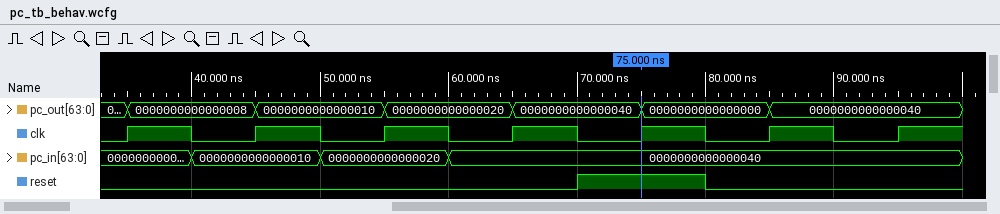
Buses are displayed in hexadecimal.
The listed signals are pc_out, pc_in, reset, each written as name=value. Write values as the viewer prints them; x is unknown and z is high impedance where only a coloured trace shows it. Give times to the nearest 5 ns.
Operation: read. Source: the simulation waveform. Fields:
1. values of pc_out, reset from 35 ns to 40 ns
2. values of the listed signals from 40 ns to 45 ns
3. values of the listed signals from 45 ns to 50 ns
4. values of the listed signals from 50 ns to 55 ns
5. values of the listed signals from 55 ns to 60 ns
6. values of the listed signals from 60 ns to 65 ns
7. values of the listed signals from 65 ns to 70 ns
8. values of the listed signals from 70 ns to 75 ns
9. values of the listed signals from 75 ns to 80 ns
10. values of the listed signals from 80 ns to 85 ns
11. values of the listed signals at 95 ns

pc_out=0000000000000008, reset=0
pc_out=0000000000000008, pc_in=0000000000000010, reset=0
pc_out=0000000000000010, pc_in=0000000000000010, reset=0
pc_out=0000000000000010, pc_in=0000000000000020, reset=0
pc_out=0000000000000020, pc_in=0000000000000020, reset=0
pc_out=0000000000000020, pc_in=0000000000000040, reset=0
pc_out=0000000000000040, pc_in=0000000000000040, reset=0
pc_out=0000000000000040, pc_in=0000000000000040, reset=1
pc_out=0000000000000000, pc_in=0000000000000040, reset=1
pc_out=0000000000000000, pc_in=0000000000000040, reset=0
pc_out=0000000000000040, pc_in=0000000000000040, reset=0
